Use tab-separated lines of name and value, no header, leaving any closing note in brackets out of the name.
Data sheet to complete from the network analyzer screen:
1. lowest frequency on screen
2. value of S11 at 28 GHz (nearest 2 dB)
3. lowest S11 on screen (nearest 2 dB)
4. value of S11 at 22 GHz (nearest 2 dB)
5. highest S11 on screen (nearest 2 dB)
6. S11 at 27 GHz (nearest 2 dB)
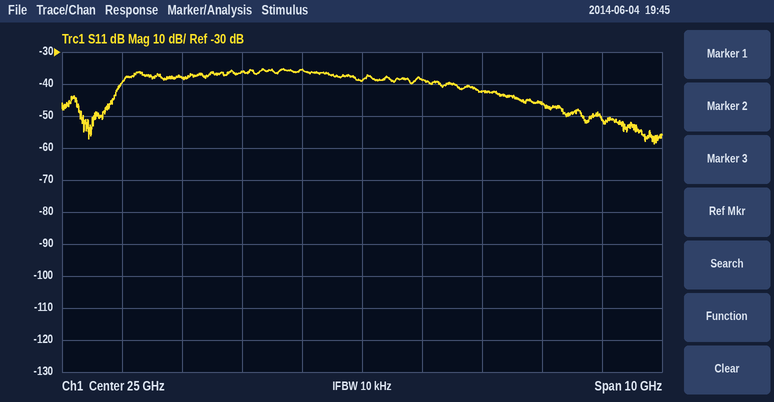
lowest frequency on screen	20 GHz
value of S11 at 28 GHz	-46 dB
lowest S11 on screen	-58 dB
value of S11 at 22 GHz	-38 dB
highest S11 on screen	-36 dB
S11 at 27 GHz	-42 dB
